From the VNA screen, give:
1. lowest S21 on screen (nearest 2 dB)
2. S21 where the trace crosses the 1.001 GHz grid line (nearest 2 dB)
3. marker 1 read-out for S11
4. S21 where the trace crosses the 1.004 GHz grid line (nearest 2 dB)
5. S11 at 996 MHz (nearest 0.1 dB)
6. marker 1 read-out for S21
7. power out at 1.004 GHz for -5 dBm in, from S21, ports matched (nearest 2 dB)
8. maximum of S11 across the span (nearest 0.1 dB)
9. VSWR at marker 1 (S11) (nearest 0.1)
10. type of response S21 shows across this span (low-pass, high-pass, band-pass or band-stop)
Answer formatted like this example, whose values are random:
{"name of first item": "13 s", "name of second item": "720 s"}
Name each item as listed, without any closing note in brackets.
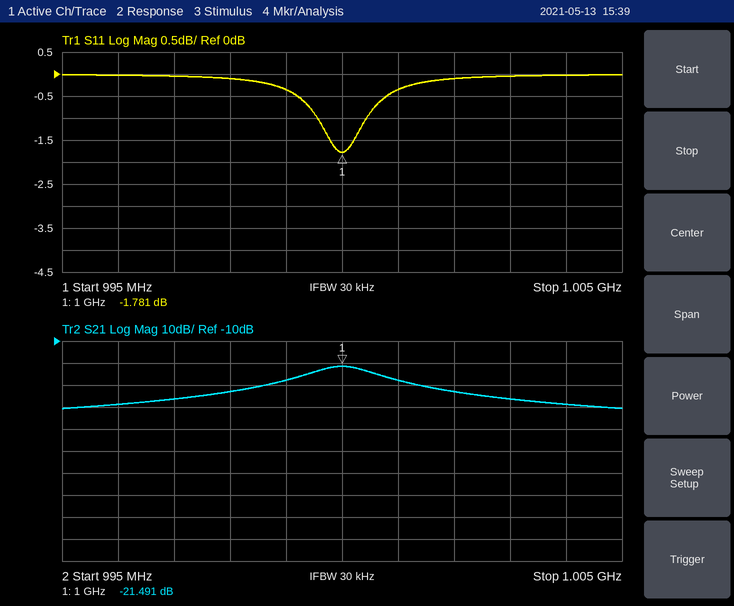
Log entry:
{"lowest S21 on screen": "-40 dB", "S21 where the trace crosses the 1.001 GHz grid line": "-28 dB", "marker 1 read-out for S11": "-1.781 dB", "S21 where the trace crosses the 1.004 GHz grid line": "-38 dB", "S11 at 996 MHz": "0.0 dB", "marker 1 read-out for S21": "-21.491 dB", "power out at 1.004 GHz for -5 dBm in, from S21, ports matched": "-44 dBm", "maximum of S11 across the span": "0.0 dB", "VSWR at marker 1 (S11)": "9.8", "type of response S21 shows across this span": "band-pass"}
